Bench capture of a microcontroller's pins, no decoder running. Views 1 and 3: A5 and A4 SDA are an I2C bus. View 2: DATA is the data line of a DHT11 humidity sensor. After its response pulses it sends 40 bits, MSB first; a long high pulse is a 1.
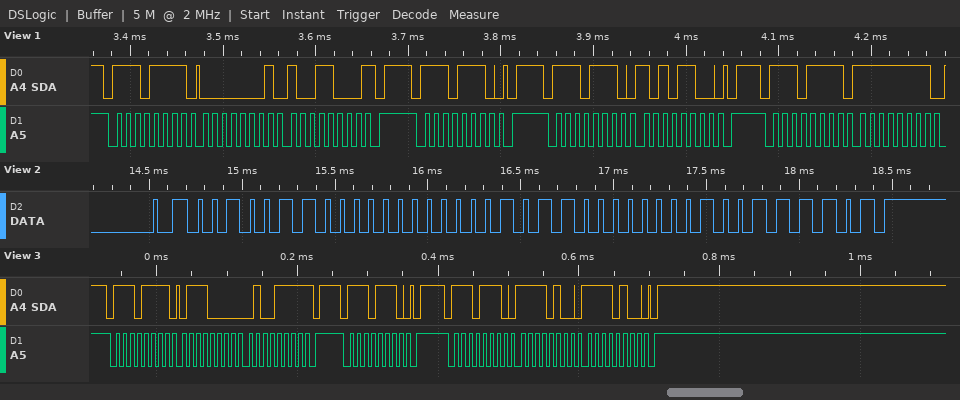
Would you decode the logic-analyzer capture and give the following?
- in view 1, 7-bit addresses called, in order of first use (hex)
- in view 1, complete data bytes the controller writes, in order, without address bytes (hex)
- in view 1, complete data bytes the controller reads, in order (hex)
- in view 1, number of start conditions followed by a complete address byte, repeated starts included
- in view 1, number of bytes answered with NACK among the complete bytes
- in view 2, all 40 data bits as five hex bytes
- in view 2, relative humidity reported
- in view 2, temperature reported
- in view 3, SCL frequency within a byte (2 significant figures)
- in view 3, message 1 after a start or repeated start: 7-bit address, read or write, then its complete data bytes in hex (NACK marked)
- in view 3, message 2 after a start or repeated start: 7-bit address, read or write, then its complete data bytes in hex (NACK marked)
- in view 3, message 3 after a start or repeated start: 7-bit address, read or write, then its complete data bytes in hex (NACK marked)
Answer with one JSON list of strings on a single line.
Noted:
["0x77", "AC", "01 98 FF", "4", "1", "26 00 16 01 3D", "38 %", "22.1 °C", "100 kHz", "0x77 read: 70 4F NACK", "0x77 write", "0x77 write: F4 F4"]
